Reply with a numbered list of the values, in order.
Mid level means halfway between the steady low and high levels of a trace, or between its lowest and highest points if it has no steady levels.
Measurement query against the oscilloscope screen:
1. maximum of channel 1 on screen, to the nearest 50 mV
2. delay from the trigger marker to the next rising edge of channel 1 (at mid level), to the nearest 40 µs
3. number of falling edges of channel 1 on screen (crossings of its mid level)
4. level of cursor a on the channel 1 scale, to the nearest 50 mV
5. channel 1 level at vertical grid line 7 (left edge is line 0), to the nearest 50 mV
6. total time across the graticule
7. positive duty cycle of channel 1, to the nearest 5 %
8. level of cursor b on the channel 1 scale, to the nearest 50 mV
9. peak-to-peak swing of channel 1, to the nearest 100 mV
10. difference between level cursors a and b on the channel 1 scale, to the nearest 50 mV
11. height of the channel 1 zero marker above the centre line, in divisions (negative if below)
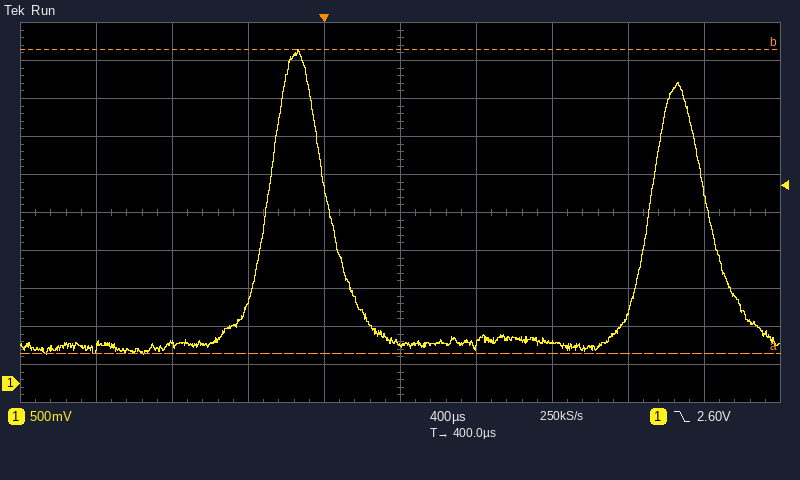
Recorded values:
1. 4.40 V
2. 1.72 ms
3. 2
4. 400 mV
5. 550 mV
6. 4 ms
7. 15 %
8. 4.40 V
9. 4.00 V
10. 4.00 V
11. -4.5 div
